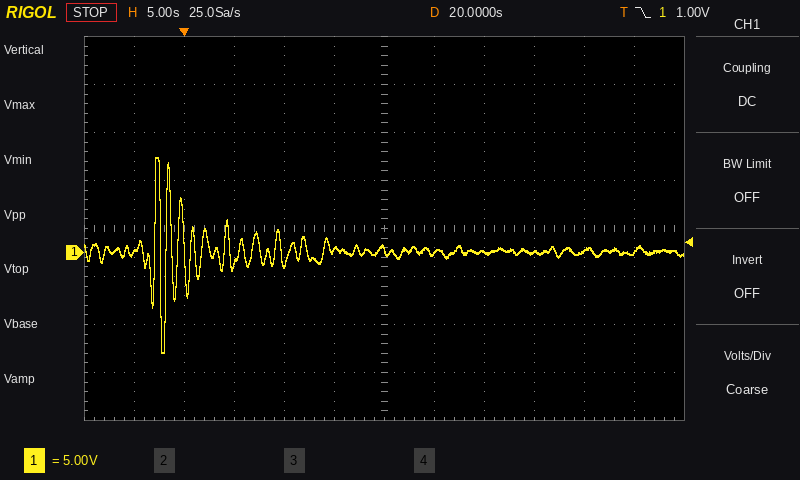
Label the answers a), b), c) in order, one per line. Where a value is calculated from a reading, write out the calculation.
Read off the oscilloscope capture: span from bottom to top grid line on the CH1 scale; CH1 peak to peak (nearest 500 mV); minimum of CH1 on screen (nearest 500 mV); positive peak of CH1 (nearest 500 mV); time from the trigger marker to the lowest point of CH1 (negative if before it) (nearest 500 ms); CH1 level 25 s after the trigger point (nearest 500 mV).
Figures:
a) 40 V
b) 10.0 V − (-10.5 V) = 20.5 V
c) -10.5 V
d) 10.0 V
e) -2.0 s
f) 0.0 V
